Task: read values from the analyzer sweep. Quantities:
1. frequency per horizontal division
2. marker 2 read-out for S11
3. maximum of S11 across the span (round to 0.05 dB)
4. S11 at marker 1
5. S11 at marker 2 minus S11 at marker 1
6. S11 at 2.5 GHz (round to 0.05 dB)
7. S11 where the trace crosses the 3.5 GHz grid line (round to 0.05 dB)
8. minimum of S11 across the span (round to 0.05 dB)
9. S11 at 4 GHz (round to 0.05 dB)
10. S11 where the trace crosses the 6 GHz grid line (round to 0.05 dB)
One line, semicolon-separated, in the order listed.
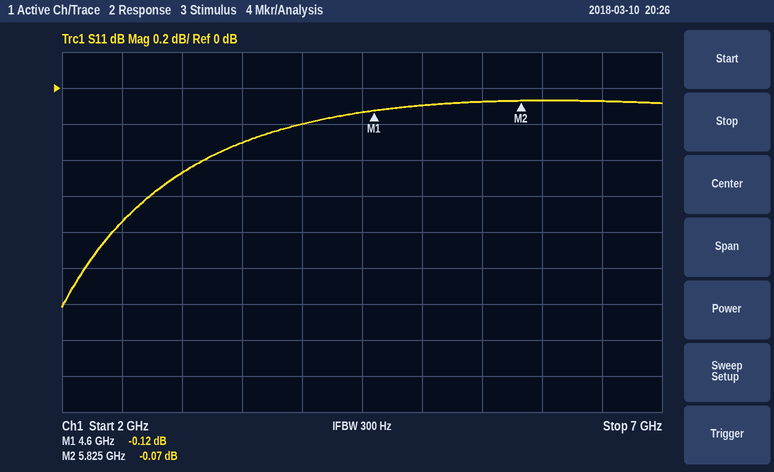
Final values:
500 MHz; -0.07 dB; -0.05 dB; -0.12 dB; 0.05 dB; -0.75 dB; -0.30 dB; -1.20 dB; -0.20 dB; -0.05 dB
